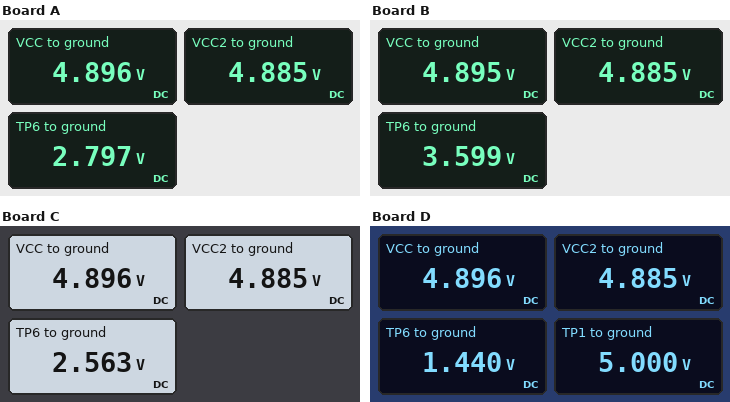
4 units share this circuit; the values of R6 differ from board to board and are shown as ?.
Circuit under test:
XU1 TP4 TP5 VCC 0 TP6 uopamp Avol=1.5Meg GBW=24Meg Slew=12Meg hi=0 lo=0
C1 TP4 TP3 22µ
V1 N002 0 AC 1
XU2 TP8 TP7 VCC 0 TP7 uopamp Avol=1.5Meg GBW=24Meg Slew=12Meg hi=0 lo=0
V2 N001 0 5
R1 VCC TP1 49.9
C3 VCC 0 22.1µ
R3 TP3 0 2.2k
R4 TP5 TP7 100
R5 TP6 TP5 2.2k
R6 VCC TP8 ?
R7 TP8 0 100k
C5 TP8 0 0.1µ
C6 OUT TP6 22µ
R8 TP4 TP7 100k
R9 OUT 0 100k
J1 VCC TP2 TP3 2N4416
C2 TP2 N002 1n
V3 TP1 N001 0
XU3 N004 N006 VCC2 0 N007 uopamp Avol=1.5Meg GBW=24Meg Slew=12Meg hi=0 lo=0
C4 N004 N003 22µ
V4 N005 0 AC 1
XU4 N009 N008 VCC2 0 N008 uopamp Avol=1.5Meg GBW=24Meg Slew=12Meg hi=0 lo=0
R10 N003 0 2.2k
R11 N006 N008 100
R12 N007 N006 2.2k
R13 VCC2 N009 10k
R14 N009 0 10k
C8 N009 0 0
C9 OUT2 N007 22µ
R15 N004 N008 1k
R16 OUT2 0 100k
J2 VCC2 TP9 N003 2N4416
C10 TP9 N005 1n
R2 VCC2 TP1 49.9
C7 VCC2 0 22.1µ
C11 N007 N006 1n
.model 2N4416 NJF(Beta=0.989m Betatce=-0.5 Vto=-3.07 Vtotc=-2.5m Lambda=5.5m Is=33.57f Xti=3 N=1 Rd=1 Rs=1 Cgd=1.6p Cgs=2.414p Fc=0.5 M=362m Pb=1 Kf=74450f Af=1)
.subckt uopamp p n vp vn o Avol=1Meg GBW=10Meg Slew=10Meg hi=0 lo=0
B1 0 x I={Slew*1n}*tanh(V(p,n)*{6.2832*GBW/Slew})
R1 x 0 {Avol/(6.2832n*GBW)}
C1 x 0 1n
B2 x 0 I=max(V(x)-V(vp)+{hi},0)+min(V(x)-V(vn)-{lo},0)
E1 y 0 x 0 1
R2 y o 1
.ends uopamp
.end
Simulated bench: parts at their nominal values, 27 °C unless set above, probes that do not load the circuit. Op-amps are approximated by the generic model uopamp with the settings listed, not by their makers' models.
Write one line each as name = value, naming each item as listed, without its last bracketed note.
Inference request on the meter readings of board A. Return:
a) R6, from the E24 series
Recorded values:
R6, from the E24 series = 75 kΩ
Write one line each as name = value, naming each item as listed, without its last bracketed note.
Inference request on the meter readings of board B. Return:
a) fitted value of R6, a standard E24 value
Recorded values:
fitted value of R6, a standard E24 value = 36 kΩ
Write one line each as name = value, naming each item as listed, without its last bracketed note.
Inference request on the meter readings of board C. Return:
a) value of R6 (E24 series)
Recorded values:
value of R6 = 91 kΩ
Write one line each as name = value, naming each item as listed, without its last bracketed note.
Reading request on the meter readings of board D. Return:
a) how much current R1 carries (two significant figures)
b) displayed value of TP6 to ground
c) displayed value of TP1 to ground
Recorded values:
how much current R1 carries = 2.1 mA
displayed value of TP6 to ground = 1.440 V
displayed value of TP1 to ground = 5.000 V
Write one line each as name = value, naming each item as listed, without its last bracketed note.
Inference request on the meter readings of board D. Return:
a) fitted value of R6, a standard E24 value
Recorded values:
fitted value of R6, a standard E24 value = 240 kΩ
